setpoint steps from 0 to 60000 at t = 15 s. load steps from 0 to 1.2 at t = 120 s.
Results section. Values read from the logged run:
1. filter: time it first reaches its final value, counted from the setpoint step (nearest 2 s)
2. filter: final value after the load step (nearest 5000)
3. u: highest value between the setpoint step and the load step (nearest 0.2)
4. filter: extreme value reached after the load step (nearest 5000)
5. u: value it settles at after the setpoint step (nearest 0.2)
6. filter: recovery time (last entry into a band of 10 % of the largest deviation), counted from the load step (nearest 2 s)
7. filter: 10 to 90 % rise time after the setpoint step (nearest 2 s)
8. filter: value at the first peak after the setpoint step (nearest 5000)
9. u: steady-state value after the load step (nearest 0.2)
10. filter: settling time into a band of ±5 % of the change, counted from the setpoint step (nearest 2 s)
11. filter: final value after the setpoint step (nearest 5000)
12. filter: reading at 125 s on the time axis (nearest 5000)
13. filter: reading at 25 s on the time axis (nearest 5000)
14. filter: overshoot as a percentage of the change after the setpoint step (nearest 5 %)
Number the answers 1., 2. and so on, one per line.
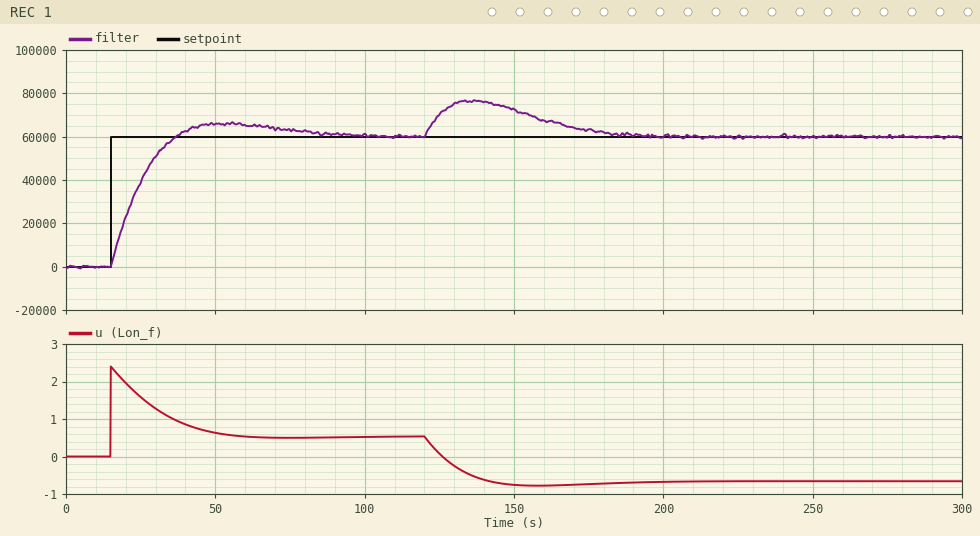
1. 22 s
2. 60000
3. 2.4
4. 75000
5. 0.6
6. 62 s
7. 16 s
8. 65000
9. -0.6
10. 60 s
11. 60000
12. 70000
13. 40000
14. 10 %
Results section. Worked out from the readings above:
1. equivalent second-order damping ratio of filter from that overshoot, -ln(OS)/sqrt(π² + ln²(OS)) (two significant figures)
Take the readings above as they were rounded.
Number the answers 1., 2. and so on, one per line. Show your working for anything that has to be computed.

1. ln(0.1) = -2.303; 2.303 / sqrt(9.870 + 5.302) = 0.59
